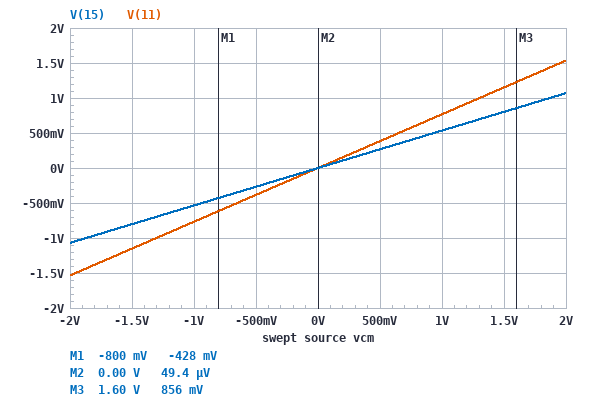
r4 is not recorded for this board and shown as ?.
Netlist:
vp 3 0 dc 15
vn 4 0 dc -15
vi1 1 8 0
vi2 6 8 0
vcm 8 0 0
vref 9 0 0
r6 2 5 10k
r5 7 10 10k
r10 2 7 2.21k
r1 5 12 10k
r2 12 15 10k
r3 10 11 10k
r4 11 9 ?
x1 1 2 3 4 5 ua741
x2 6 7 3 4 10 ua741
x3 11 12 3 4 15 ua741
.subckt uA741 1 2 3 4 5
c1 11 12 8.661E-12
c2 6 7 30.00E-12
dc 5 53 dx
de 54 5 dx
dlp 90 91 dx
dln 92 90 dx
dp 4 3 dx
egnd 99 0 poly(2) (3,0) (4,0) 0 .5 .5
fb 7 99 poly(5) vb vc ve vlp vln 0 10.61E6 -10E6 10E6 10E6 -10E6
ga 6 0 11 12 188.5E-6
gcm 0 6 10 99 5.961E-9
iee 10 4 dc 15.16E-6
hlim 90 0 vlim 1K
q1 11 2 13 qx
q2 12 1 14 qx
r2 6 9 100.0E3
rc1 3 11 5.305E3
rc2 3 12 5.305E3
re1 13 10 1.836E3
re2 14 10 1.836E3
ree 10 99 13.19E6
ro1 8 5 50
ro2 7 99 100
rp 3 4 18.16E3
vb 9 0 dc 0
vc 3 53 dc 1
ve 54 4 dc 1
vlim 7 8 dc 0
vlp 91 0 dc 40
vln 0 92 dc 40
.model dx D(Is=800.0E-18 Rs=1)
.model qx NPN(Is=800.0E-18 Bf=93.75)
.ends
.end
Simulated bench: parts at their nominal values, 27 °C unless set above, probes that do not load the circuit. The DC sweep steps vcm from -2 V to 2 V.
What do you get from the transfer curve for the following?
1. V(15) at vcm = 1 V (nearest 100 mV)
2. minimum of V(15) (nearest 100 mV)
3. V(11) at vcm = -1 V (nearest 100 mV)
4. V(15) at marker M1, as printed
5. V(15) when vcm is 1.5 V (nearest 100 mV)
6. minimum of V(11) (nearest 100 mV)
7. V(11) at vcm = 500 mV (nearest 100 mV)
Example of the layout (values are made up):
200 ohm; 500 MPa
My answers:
500 mV; -1.1 V; -800 mV; -428 mV; 800 mV; -1.5 V; 400 mV
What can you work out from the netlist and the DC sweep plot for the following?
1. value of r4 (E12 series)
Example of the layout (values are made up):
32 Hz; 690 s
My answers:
33 kΩ
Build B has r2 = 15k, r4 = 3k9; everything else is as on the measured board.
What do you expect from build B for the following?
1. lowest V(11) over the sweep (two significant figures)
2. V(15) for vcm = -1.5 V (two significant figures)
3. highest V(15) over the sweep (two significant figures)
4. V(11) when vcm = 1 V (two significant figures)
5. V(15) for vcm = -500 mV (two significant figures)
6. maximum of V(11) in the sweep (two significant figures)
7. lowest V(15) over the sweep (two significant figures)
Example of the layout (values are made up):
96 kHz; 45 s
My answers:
-560 mV; 1.2 V; 1.6 V; 280 mV; 400 mV; 560 mV; -1.6 V
